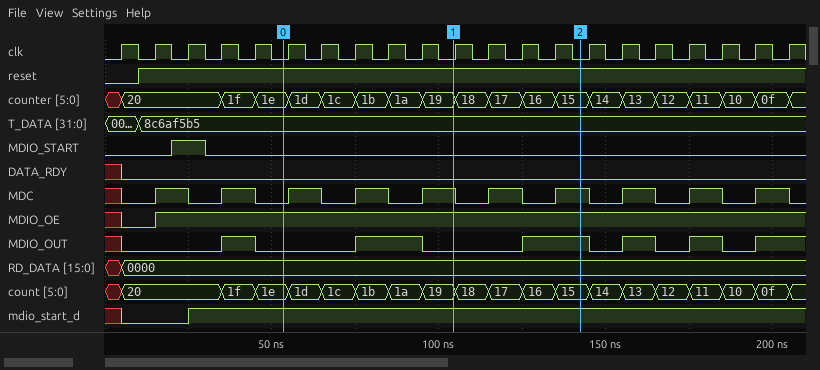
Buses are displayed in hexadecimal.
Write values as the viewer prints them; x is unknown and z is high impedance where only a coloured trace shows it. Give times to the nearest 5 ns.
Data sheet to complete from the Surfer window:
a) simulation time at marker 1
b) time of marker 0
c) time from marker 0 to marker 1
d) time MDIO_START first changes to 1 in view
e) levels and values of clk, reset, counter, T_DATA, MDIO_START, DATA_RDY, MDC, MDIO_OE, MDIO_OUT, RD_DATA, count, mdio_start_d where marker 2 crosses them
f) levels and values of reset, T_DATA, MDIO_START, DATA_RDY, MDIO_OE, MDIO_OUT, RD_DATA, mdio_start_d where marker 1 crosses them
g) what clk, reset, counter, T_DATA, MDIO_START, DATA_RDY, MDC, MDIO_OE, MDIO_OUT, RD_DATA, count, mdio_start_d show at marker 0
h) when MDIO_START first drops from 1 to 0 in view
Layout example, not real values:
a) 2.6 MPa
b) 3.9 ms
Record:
a) 105 ns
b) 55 ns
c) 50 ns
d) 20 ns
e) clk=0, reset=1, counter=15, T_DATA=8c6af5b5, MDIO_START=0, DATA_RDY=0, MDC=1, MDIO_OE=1, MDIO_OUT=1, RD_DATA=0000, count=15, mdio_start_d=1
f) reset=1, T_DATA=8c6af5b5, MDIO_START=0, DATA_RDY=0, MDIO_OE=1, MDIO_OUT=0, RD_DATA=0000, mdio_start_d=1
g) clk=0, reset=1, counter=1e, T_DATA=8c6af5b5, MDIO_START=0, DATA_RDY=0, MDC=0, MDIO_OE=1, MDIO_OUT=0, RD_DATA=0000, count=1e, mdio_start_d=1
h) 30 ns
